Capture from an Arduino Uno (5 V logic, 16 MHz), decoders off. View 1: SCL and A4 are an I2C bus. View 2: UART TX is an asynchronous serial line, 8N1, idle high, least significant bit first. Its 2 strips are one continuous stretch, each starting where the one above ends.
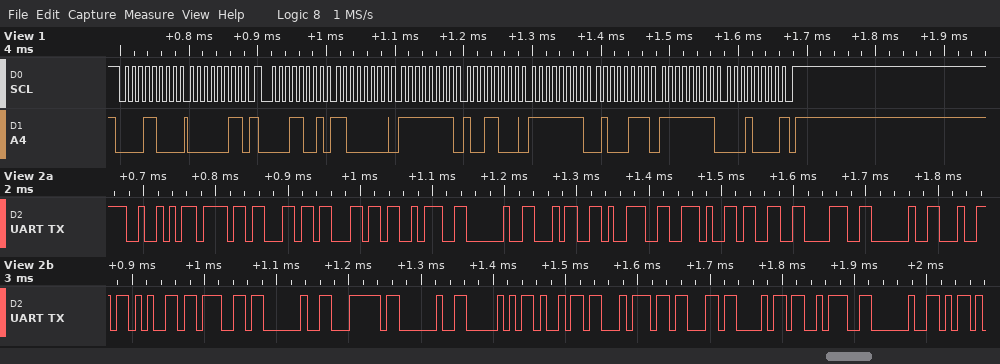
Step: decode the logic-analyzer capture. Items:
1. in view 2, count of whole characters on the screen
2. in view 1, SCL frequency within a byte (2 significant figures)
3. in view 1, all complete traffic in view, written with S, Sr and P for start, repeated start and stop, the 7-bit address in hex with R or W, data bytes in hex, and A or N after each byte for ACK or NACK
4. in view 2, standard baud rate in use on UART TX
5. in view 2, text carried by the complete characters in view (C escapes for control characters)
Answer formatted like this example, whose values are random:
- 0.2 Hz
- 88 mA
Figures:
- 25
- 100 kHz
- S 0CW A 03 A Sr 0CR A C0 A FF A 98 A FF A 47 A FF A 10 N P
- 115200 baud
- "Roll: 49.38 deg | Pitch: "
